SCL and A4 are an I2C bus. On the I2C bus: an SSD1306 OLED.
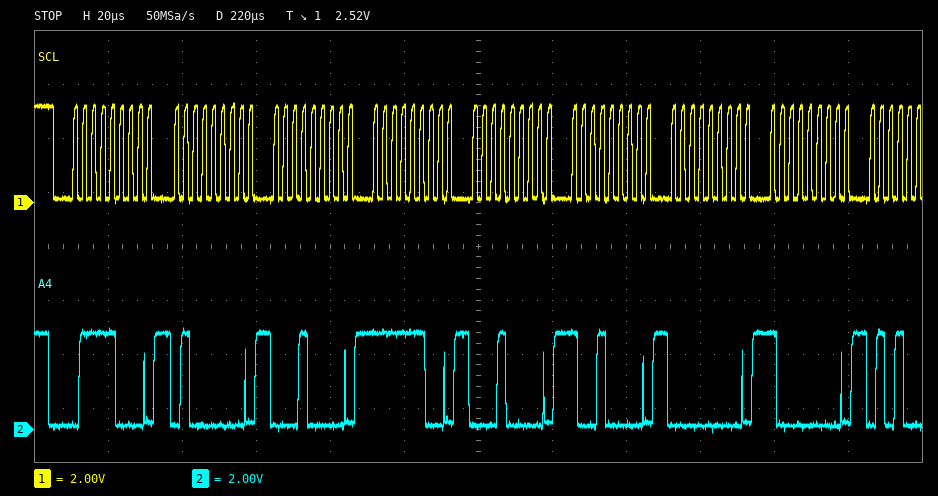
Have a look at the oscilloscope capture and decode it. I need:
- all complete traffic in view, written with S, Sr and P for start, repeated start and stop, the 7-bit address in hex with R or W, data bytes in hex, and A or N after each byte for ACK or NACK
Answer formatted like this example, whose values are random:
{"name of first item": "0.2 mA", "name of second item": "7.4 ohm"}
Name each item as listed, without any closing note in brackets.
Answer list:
{"all complete traffic in view, written with S, Sr and P for start, repeated start and stop, the 7-bit address in hex with R or W, data bytes in hex, and A or N after each byte for ACK or NACK": "S 3CW A 40 A 10 A FC A 10 A 90 A 00 A 80 A"}
